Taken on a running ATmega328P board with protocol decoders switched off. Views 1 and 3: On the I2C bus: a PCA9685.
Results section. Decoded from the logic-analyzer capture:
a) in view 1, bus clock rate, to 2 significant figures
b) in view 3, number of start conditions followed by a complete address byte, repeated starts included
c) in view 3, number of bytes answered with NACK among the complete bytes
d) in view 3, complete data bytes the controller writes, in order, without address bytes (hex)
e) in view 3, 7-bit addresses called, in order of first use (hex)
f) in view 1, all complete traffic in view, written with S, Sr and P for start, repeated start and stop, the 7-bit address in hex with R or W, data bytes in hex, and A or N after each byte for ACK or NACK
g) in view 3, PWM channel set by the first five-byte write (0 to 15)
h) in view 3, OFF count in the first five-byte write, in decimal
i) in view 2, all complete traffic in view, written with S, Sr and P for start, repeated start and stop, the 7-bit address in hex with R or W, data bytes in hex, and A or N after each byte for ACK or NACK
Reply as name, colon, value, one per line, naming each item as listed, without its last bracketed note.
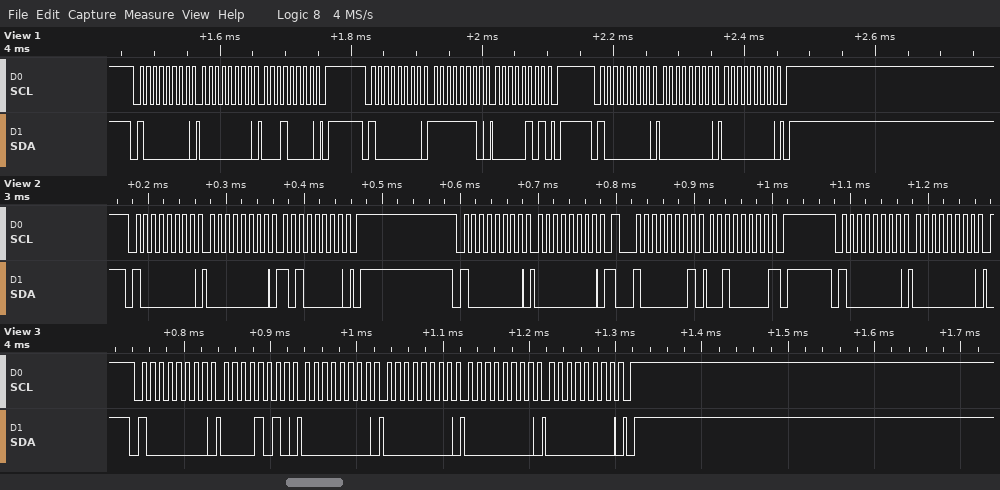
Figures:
in view 1, bus clock rate, to 2 significant figures: 100 kHz
in view 3, number of start conditions followed by a complete address byte, repeated starts included: 1
in view 3, number of bytes answered with NACK among the complete bytes: 0
in view 3, complete data bytes the controller writes, in order, without address bytes: 0A 00 00 00 00
in view 3, 7-bit addresses called, in order of first use: 0x40
in view 1, all complete traffic in view, written with S, Sr and P for start, repeated start and stop, the 7-bit address in hex with R or W, data bytes in hex, and A or N after each byte for ACK or NACK: S 40W A 00 A 10 A P S 40W A FE A 05 A P S 40W A 00 A 00 A P
in view 3, PWM channel set by the first five-byte write: 1
in view 3, OFF count in the first five-byte write, in decimal: 0
in view 2, all complete traffic in view, written with S, Sr and P for start, repeated start and stop, the 7-bit address in hex with R or W, data bytes in hex, and A or N after each byte for ACK or NACK: S 40W A 00 A A0 A P S 40W A 00 A Sr 40R A 20 N P S 40W A 00 A
